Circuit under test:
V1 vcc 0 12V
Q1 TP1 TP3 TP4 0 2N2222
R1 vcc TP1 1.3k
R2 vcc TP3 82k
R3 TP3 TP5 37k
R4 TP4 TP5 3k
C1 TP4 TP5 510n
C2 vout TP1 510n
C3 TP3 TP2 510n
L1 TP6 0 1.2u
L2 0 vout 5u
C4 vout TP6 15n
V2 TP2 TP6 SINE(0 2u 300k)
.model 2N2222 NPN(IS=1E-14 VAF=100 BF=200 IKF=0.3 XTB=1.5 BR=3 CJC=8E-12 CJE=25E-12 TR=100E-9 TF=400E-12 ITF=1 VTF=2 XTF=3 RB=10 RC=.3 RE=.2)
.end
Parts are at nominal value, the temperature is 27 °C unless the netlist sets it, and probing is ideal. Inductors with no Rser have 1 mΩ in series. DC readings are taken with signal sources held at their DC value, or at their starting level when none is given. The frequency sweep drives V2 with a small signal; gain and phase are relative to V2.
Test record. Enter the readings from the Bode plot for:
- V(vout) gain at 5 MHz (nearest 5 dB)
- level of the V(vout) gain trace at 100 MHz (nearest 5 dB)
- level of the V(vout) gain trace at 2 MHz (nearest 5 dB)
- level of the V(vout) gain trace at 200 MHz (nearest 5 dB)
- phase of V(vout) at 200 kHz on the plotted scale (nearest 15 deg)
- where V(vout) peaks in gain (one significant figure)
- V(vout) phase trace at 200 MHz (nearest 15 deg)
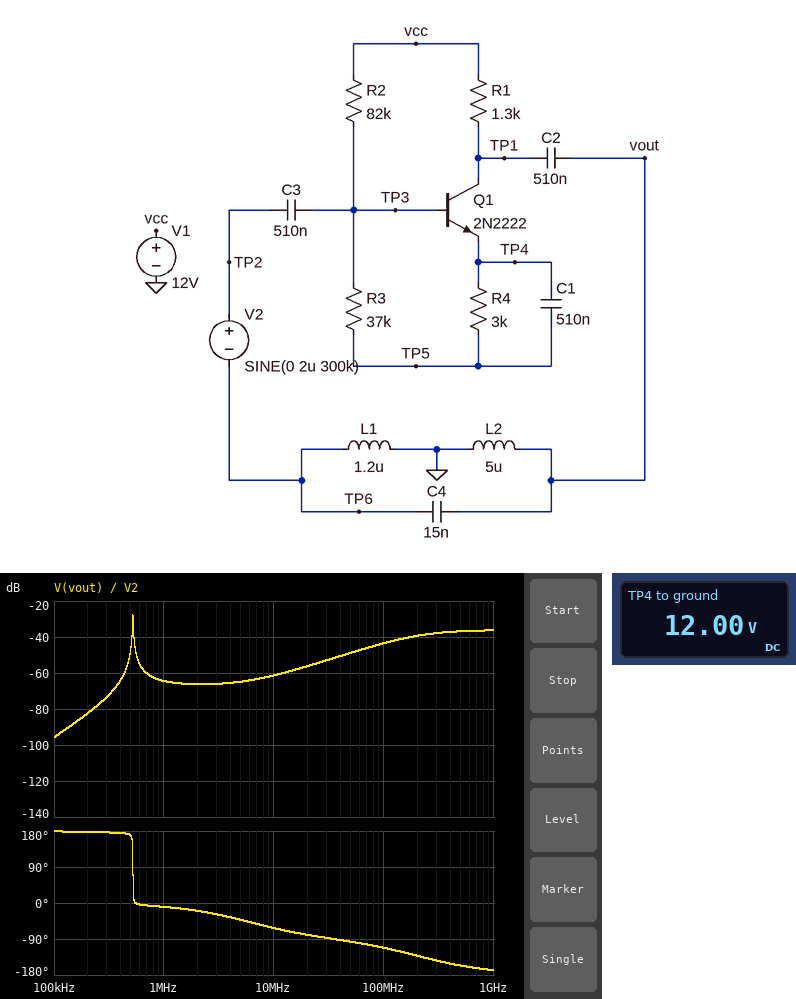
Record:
-65 dB
-45 dB
-65 dB
-40 dB
180 deg
500 kHz
-135 deg
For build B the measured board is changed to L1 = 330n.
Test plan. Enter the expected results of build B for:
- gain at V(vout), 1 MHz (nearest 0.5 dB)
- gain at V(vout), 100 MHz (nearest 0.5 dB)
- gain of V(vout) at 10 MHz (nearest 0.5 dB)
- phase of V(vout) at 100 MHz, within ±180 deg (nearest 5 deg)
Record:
-62.5 dB
-52.5 dB
-65.0 dB
-85 deg
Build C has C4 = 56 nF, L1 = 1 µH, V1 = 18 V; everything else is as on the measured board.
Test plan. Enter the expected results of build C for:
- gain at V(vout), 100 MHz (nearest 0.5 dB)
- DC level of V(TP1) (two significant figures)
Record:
-44.5 dB
18 V
